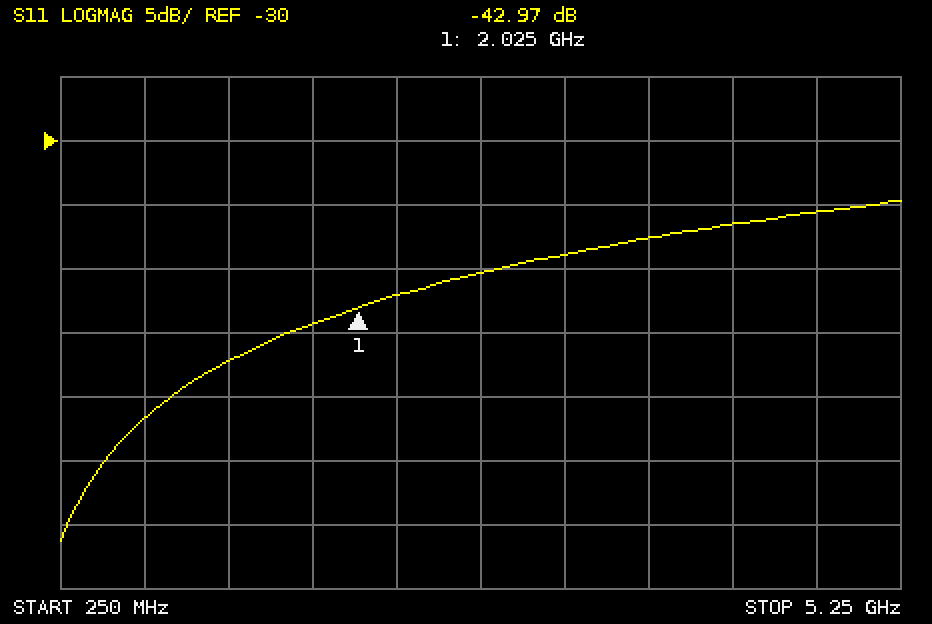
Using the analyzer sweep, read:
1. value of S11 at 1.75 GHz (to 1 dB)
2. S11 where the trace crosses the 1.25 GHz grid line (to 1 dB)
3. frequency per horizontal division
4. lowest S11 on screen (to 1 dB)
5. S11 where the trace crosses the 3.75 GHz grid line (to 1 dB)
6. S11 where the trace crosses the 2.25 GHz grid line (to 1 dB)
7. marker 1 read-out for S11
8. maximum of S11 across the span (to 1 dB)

-44 dB
-47 dB
500 MHz
-61 dB
-38 dB
-42 dB
-42.97 dB
-35 dB
